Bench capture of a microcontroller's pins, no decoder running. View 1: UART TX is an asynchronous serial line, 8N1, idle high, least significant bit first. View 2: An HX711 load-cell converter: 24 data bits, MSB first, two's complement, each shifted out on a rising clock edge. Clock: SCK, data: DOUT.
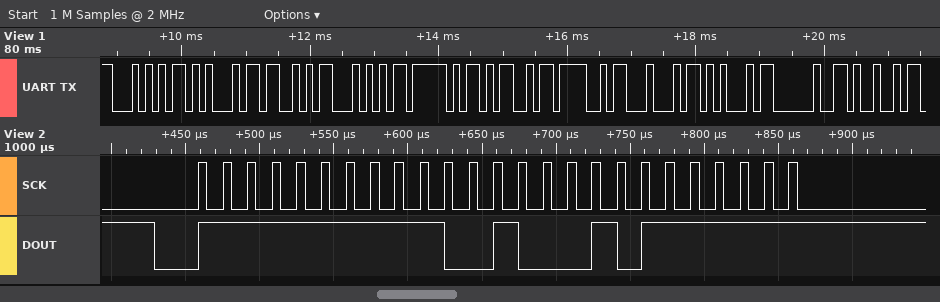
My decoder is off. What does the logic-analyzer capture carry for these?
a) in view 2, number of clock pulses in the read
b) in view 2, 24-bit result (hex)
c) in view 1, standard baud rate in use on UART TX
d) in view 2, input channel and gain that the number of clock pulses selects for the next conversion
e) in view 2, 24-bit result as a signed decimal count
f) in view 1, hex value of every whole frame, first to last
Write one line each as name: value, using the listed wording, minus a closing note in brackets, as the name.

in view 2, number of clock pulses in the read: 25
in view 2, 24-bit result: 0xFFC8BF
in view 1, standard baud rate in use on UART TX: 9600 baud
in view 2, input channel and gain that the number of clock pulses selects for the next conversion: channel A, gain 128
in view 2, 24-bit result as a signed decimal count: -14145
in view 1, hex value of every whole frame, first to last: 0x54 0x45 0x53 0x54 0x5F 0x4D 0x4F 0x44 0x45 0x20 0x49
